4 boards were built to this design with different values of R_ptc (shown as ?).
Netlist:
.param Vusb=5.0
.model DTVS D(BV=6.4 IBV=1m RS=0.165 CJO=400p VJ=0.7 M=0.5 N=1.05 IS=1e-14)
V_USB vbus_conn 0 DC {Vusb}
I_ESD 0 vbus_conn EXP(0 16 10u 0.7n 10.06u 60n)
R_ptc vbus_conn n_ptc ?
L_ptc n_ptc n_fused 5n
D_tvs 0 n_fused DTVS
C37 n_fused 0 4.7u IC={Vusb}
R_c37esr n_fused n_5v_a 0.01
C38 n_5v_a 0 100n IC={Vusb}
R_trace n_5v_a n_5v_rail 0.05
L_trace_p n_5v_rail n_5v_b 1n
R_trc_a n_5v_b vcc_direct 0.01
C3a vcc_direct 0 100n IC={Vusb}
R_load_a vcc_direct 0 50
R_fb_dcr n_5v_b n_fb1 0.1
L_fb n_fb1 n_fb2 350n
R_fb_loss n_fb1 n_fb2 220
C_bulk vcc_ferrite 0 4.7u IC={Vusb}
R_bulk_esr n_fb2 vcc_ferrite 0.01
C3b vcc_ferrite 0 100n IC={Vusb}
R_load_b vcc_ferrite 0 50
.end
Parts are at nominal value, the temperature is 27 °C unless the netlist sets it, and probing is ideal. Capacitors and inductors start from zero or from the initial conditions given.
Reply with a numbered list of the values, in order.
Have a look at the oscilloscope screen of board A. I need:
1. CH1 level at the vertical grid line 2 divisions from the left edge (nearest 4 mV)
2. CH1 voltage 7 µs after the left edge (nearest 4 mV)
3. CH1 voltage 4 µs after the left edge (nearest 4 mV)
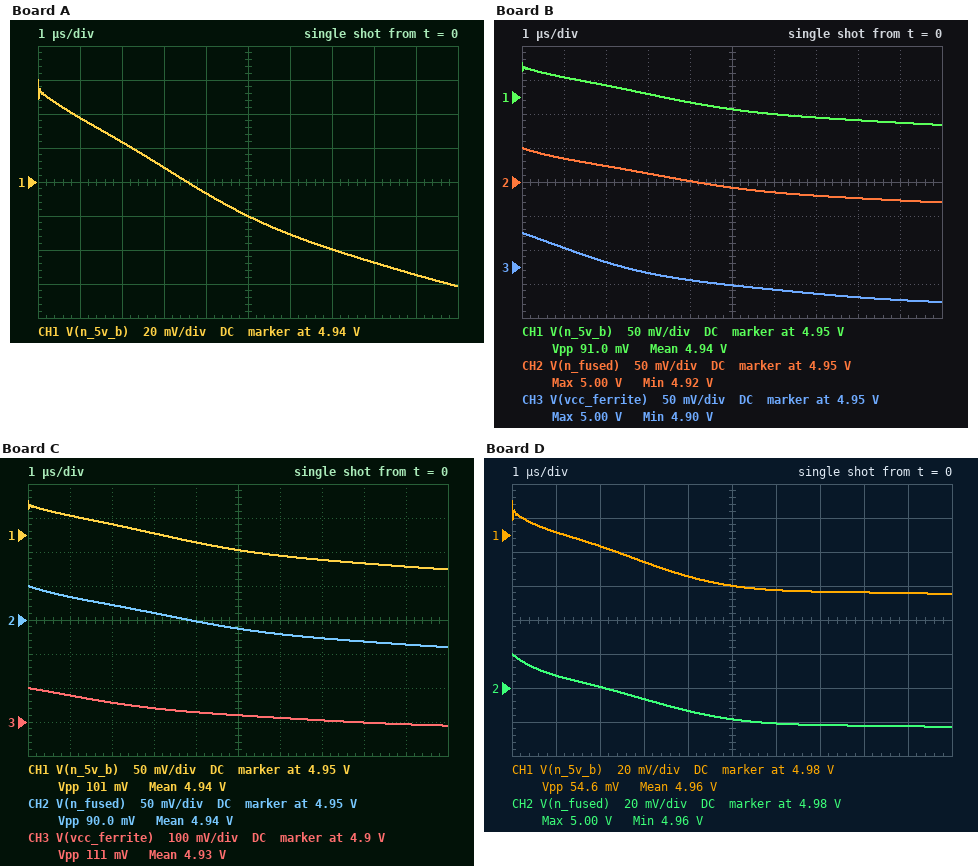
1. 4.964 V
2. 4.900 V
3. 4.932 V
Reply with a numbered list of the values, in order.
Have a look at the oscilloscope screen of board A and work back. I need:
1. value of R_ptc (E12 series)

1. 0.82 Ω
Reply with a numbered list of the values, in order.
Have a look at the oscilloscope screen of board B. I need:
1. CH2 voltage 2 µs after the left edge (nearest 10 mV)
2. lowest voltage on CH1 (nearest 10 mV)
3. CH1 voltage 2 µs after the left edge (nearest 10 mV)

1. 4.97 V
2. 4.91 V
3. 4.97 V
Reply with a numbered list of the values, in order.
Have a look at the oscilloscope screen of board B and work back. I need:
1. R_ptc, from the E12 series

1. 0.47 Ω
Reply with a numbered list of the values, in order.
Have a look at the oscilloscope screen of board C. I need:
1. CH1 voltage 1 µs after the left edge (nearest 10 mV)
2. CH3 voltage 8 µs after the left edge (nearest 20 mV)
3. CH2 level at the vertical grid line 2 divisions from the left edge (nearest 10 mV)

1. 4.98 V
2. 4.90 V
3. 4.97 V
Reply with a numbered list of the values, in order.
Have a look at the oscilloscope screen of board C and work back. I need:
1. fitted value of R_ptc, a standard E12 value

1. 0.56 Ω
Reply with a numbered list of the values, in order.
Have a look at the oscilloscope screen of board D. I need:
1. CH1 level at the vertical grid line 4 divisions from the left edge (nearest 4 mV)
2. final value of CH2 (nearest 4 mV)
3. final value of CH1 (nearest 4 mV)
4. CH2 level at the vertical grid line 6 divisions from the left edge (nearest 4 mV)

1. 4.956 V
2. 4.956 V
3. 4.944 V
4. 4.960 V
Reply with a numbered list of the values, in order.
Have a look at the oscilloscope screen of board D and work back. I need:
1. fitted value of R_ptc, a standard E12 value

1. 0.22 Ω
